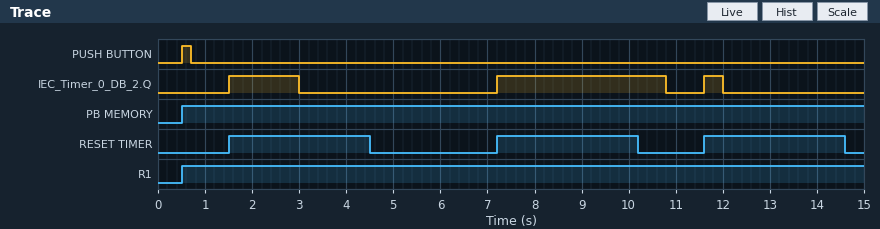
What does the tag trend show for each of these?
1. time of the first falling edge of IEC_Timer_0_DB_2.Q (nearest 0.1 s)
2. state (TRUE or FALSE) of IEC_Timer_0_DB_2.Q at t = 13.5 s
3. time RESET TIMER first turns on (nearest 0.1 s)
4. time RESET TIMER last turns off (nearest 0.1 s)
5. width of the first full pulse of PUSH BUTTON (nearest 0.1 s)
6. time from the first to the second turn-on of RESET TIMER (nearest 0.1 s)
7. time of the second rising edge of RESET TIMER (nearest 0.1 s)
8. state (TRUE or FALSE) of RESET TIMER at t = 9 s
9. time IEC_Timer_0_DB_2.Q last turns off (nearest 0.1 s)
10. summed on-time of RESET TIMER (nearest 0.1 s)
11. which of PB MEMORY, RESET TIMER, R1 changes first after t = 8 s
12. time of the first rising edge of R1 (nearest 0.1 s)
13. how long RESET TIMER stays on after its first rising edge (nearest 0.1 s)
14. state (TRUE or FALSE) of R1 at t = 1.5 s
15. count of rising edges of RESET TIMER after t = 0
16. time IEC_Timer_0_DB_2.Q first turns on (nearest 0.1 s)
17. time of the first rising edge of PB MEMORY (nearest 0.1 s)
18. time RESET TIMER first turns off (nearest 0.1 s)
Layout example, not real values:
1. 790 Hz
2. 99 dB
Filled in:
1. 3.0 s
2. FALSE
3. 1.5 s
4. 14.6 s
5. 0.2 s
6. 5.7 s
7. 7.2 s
8. TRUE
9. 12.0 s
10. 9.0 s
11. RESET TIMER
12. 0.5 s
13. 3.0 s
14. TRUE
15. 3
16. 1.5 s
17. 0.5 s
18. 4.5 s
